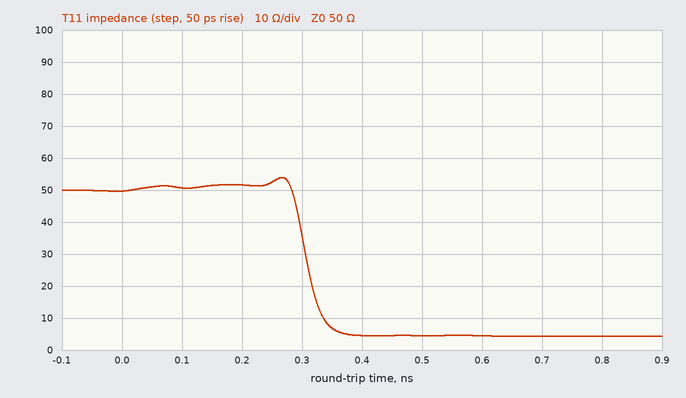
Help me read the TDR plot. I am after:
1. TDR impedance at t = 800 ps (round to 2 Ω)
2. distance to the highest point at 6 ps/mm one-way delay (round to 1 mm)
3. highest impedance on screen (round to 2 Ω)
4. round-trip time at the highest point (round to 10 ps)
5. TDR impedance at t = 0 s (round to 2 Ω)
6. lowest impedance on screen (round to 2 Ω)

4 Ω
22 mm
54 Ω
270 ps
50 Ω
4 Ω
